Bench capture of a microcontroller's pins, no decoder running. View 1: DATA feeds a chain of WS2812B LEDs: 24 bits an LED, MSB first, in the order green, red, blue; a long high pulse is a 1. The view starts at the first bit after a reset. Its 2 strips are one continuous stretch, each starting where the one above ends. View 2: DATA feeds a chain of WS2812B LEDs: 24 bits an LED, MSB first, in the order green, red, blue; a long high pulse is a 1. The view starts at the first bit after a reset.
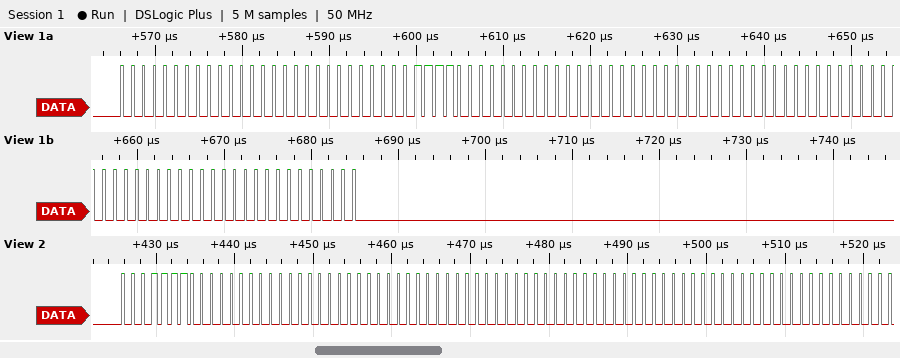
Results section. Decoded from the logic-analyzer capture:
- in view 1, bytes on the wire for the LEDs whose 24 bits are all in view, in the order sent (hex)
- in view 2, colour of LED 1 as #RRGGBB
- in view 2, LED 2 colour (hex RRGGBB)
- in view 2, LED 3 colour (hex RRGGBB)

00 00 00 1E 00 00 00 00 00 00 00 00
#001E00
#000000
#000000
